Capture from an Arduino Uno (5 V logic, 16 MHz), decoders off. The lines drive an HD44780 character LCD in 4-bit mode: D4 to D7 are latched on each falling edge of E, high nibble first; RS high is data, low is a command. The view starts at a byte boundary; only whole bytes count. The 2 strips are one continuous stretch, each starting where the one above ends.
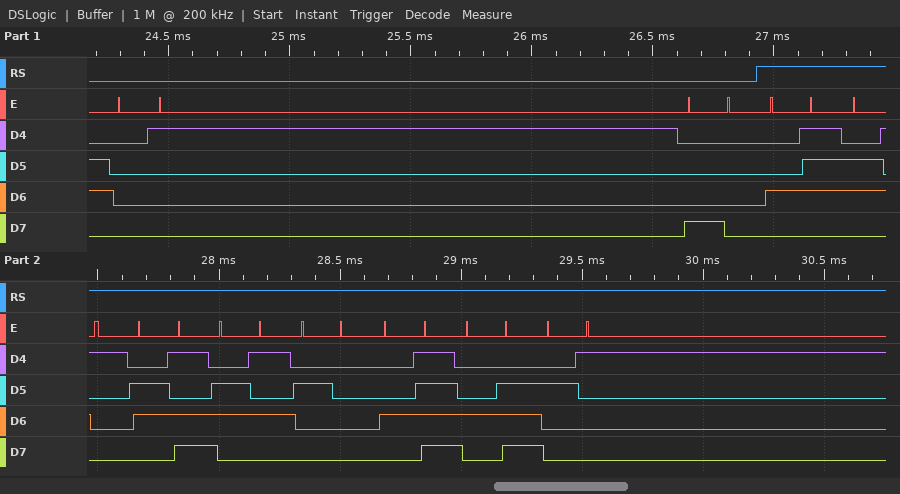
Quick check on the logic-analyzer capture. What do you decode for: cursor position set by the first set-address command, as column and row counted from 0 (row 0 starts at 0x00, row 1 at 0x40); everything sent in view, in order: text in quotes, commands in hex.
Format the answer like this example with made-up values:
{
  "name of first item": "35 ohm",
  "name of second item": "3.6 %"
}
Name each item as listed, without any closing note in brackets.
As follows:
{
  "cursor position set by the first set-address command, as column and row counted from 0": "column 0, row 0",
  "everything sent in view, in order: text in quotes, commands in hex": "0x01 0x80 \"Game ON!\""
}
